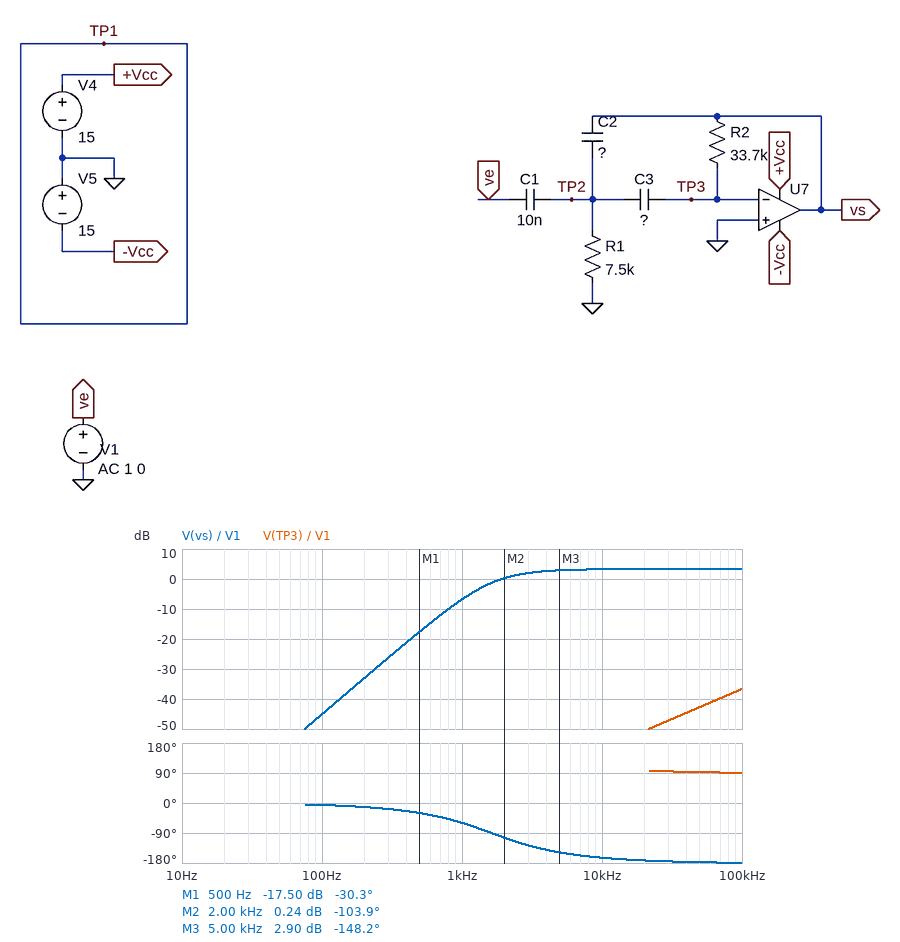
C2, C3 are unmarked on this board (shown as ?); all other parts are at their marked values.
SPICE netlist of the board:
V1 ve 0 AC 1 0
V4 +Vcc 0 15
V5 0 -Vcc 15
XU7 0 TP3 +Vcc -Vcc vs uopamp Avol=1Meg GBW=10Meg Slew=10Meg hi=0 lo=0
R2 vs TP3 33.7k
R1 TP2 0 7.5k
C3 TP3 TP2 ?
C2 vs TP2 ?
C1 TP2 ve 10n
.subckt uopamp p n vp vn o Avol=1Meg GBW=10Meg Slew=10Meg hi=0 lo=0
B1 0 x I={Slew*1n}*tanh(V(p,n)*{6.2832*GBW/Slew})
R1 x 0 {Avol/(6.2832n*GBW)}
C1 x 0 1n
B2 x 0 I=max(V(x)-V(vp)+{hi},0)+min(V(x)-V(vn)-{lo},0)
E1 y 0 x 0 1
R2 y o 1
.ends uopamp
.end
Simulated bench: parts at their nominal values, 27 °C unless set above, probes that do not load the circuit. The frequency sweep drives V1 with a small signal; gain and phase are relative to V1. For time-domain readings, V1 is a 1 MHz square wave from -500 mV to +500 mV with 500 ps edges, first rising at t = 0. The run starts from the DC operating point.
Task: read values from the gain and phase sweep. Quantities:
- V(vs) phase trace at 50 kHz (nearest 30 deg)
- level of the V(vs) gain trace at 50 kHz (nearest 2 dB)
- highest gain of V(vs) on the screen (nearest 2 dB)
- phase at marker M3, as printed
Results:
-180 deg
4 dB
4 dB
-148.2 deg
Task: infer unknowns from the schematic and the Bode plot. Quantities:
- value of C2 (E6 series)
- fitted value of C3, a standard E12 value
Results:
6.8 nF
5.6 nF
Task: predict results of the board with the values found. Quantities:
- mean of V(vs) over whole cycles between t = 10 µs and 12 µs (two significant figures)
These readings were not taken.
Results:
-600 mV
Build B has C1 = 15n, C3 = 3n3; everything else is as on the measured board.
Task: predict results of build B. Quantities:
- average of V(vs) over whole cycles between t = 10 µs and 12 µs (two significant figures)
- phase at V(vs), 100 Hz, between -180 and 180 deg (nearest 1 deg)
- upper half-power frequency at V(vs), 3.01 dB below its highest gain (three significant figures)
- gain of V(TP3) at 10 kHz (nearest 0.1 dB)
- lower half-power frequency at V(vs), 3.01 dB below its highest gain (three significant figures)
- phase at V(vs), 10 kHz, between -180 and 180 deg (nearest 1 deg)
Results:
-760 mV
-7 deg
3.85 MHz
-53.9 dB
4.46 kHz
-151 deg
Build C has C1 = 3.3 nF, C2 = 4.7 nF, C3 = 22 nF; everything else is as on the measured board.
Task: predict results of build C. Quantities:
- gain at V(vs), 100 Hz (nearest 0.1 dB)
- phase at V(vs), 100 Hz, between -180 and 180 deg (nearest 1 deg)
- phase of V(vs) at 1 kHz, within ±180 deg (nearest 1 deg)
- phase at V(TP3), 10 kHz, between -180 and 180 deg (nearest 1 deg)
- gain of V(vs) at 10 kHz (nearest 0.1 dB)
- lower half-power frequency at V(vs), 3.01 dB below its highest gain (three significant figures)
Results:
-42.8 dB
-8 deg
-91 deg
98 deg
-3.1 dB
969 Hz
